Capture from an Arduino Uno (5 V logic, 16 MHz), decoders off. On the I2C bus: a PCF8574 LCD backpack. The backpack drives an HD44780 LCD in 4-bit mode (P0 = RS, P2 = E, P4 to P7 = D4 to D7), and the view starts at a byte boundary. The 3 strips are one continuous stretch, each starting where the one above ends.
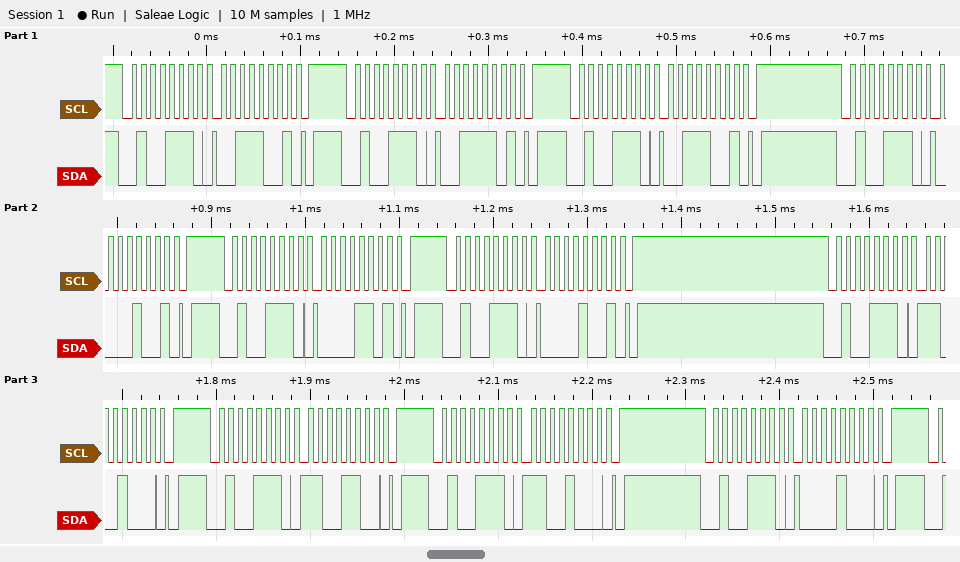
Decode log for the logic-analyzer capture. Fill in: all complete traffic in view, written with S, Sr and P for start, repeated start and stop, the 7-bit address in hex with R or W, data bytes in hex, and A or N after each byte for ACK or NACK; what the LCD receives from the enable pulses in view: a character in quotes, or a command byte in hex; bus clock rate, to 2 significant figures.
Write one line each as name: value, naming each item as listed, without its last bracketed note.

all complete traffic in view, written with S, Sr and P for start, repeated start and stop, the 7-bit address in hex with R or W, data bytes in hex, and A or N after each byte for ACK or NACK: S 27W A 39 A P S 27W A 3D A P S 27W A 39 A P S 27W A 09 A P S 27W A 0D A P S 27W A 09 A P S 27W A C8 A P S 27W A CC A P S 27W A C8 A P S 27W A 08 A P
what the LCD receives from the enable pulses in view: a character in quotes, or a command byte in hex: '0'
bus clock rate, to 2 significant figures: 100 kHz
